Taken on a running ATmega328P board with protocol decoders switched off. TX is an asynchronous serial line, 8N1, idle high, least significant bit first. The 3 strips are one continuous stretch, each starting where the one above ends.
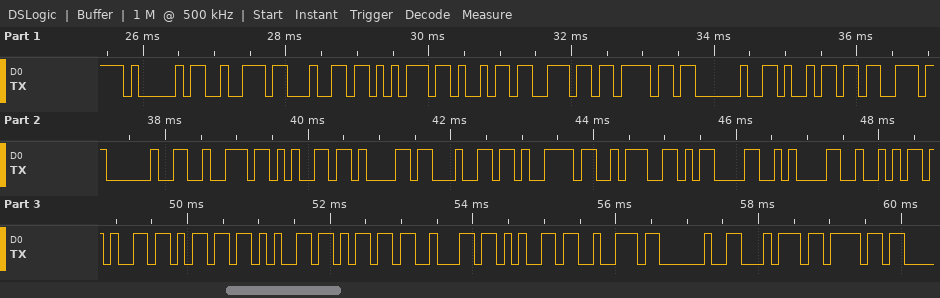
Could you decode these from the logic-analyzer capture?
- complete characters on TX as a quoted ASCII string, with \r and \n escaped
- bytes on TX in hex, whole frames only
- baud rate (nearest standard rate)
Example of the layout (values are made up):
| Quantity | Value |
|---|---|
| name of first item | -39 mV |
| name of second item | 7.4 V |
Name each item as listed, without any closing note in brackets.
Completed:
| Quantity | Value |
|---|---|
| complete characters on TX as a quoted ASCII string, with \r and \n escaped | "Arduino is ready:\r\nRemember to" |
| bytes on TX in hex, whole frames only | 41 72 64 75 69 6E 6F 20 69 73 20 72 65 61 64 79 3A 0D 0A 52 65 6D 65 6D 62 65 72 20 74 6F |
| baud rate | 9600 baud |
